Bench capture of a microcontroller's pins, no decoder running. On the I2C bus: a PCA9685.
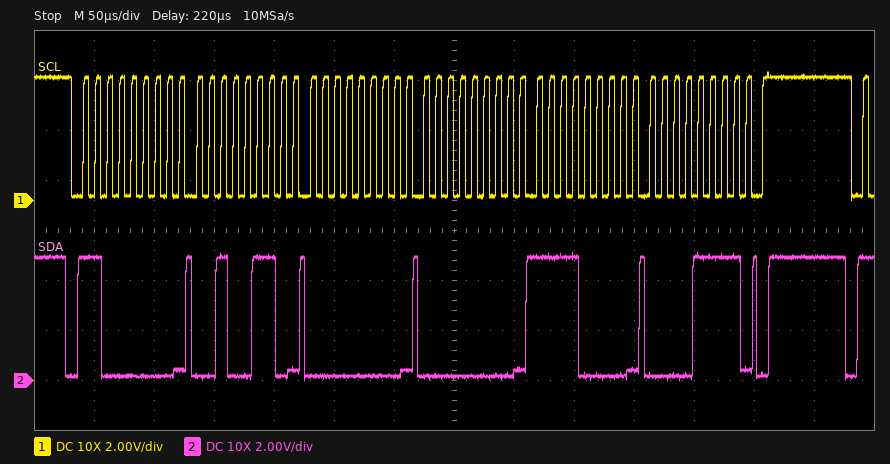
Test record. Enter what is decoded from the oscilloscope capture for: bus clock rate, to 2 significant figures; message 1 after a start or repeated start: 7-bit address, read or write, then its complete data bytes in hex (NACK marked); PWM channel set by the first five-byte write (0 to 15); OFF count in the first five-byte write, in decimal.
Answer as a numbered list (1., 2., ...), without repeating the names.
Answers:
1. 100 kHz
2. 0x60 write: 26 00 00 F0 0F
3. 8
4. 4080
